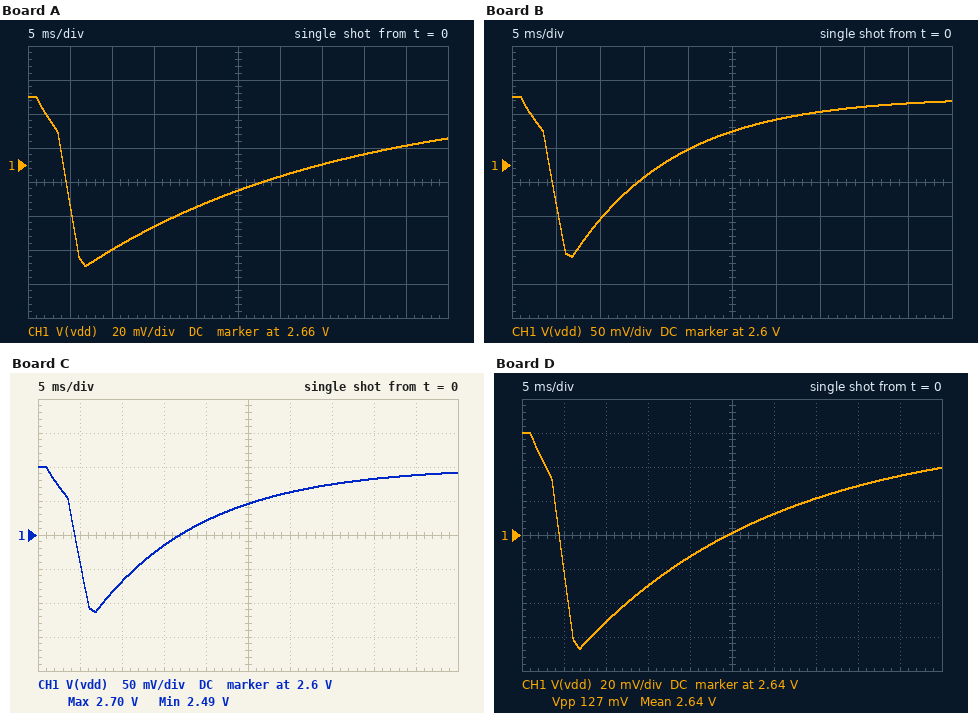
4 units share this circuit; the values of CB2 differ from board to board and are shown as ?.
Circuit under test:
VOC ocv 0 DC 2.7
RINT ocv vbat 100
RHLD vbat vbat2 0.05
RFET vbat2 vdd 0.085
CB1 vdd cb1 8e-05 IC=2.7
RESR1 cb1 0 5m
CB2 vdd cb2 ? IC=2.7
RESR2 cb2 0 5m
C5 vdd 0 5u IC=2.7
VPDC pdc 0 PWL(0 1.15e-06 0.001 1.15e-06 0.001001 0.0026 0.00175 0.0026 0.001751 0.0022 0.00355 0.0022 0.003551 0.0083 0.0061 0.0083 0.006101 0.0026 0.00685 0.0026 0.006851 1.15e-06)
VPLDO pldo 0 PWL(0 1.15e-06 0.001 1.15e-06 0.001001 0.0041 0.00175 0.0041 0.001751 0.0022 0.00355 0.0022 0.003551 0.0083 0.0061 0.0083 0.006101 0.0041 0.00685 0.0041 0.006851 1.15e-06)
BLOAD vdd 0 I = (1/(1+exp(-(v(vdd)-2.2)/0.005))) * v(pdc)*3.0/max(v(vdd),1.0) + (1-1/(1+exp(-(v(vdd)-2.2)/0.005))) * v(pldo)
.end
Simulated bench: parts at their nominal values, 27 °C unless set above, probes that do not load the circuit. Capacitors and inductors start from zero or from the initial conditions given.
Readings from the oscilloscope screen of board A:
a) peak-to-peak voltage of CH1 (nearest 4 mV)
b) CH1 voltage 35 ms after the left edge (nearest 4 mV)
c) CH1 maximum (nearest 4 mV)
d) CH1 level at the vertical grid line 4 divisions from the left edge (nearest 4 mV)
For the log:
100 mV
2.660 V
2.700 V
2.636 V
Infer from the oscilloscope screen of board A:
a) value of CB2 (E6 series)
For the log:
220 µF
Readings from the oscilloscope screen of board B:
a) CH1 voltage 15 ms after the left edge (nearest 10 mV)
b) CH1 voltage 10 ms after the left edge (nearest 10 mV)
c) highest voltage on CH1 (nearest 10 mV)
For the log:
2.58 V
2.52 V
2.70 V
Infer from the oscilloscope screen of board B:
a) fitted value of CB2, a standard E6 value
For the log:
33 µF
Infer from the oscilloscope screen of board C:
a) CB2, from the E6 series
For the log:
47 µF
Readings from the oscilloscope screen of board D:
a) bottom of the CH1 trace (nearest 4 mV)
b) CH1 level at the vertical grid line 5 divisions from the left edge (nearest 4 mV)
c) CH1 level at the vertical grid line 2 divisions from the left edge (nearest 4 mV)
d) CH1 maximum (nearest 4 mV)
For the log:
2.572 V
2.640 V
2.588 V
2.700 V
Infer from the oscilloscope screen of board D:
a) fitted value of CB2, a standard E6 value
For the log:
150 µF
